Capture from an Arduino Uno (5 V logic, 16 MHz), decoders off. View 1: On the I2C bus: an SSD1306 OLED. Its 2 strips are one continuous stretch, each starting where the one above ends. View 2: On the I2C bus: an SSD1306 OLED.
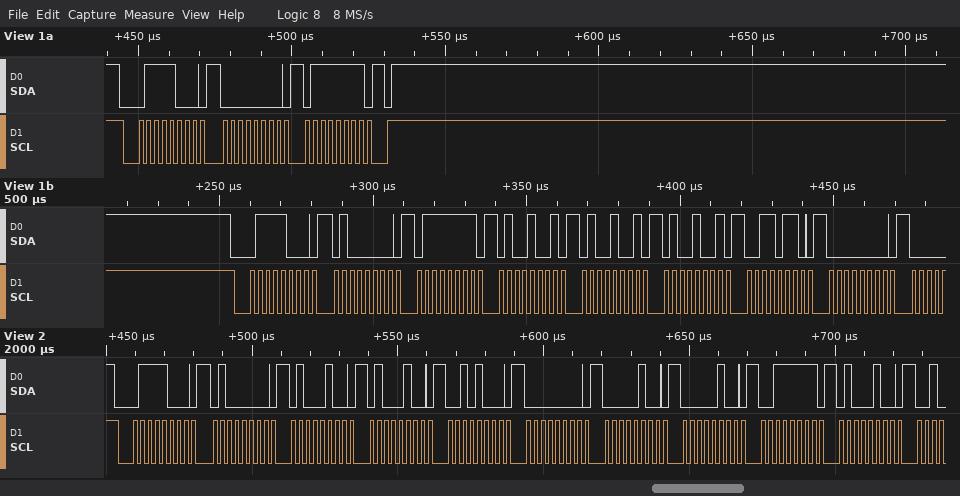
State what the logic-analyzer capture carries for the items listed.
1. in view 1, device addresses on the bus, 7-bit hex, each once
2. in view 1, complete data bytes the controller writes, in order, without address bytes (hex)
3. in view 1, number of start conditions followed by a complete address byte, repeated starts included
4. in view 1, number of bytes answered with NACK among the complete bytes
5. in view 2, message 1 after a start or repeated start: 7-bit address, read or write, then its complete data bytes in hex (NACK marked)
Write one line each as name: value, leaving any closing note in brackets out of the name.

in view 1, device addresses on the bus, 7-bit hex, each once: 0x3C
in view 1, complete data bytes the controller writes, in order, without address bytes: 00 7F 40 7F 49 49 49 36 00
in view 1, number of start conditions followed by a complete address byte, repeated starts included: 2
in view 1, number of bytes answered with NACK among the complete bytes: 0
in view 2, message 1 after a start or repeated start: 7-bit address, read or write, then its complete data bytes in hex: 0x3C write: 40 44 44 28 00 04 04 3F 44
